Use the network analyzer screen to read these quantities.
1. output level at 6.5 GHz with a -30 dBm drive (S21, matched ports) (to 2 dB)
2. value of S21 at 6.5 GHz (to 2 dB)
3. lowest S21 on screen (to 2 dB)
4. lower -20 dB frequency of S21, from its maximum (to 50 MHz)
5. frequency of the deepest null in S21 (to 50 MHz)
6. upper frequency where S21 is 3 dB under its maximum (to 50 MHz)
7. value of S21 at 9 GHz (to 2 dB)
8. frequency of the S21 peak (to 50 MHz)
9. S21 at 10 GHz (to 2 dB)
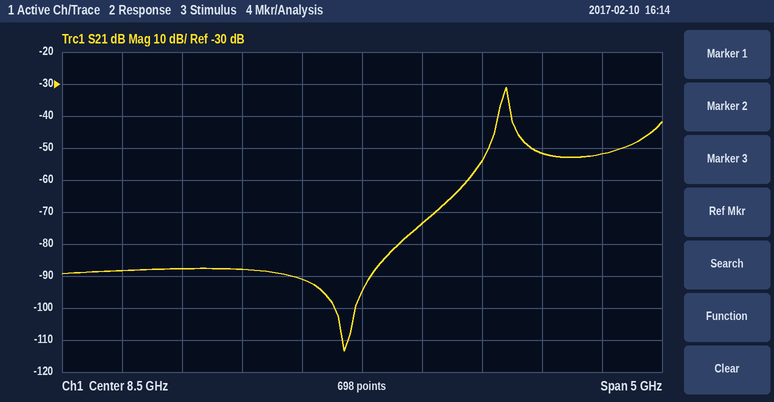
-118 dBm
-88 dB
-114 dB
9.55 GHz
8.35 GHz
9.70 GHz
-74 dB
9.70 GHz
-52 dB
